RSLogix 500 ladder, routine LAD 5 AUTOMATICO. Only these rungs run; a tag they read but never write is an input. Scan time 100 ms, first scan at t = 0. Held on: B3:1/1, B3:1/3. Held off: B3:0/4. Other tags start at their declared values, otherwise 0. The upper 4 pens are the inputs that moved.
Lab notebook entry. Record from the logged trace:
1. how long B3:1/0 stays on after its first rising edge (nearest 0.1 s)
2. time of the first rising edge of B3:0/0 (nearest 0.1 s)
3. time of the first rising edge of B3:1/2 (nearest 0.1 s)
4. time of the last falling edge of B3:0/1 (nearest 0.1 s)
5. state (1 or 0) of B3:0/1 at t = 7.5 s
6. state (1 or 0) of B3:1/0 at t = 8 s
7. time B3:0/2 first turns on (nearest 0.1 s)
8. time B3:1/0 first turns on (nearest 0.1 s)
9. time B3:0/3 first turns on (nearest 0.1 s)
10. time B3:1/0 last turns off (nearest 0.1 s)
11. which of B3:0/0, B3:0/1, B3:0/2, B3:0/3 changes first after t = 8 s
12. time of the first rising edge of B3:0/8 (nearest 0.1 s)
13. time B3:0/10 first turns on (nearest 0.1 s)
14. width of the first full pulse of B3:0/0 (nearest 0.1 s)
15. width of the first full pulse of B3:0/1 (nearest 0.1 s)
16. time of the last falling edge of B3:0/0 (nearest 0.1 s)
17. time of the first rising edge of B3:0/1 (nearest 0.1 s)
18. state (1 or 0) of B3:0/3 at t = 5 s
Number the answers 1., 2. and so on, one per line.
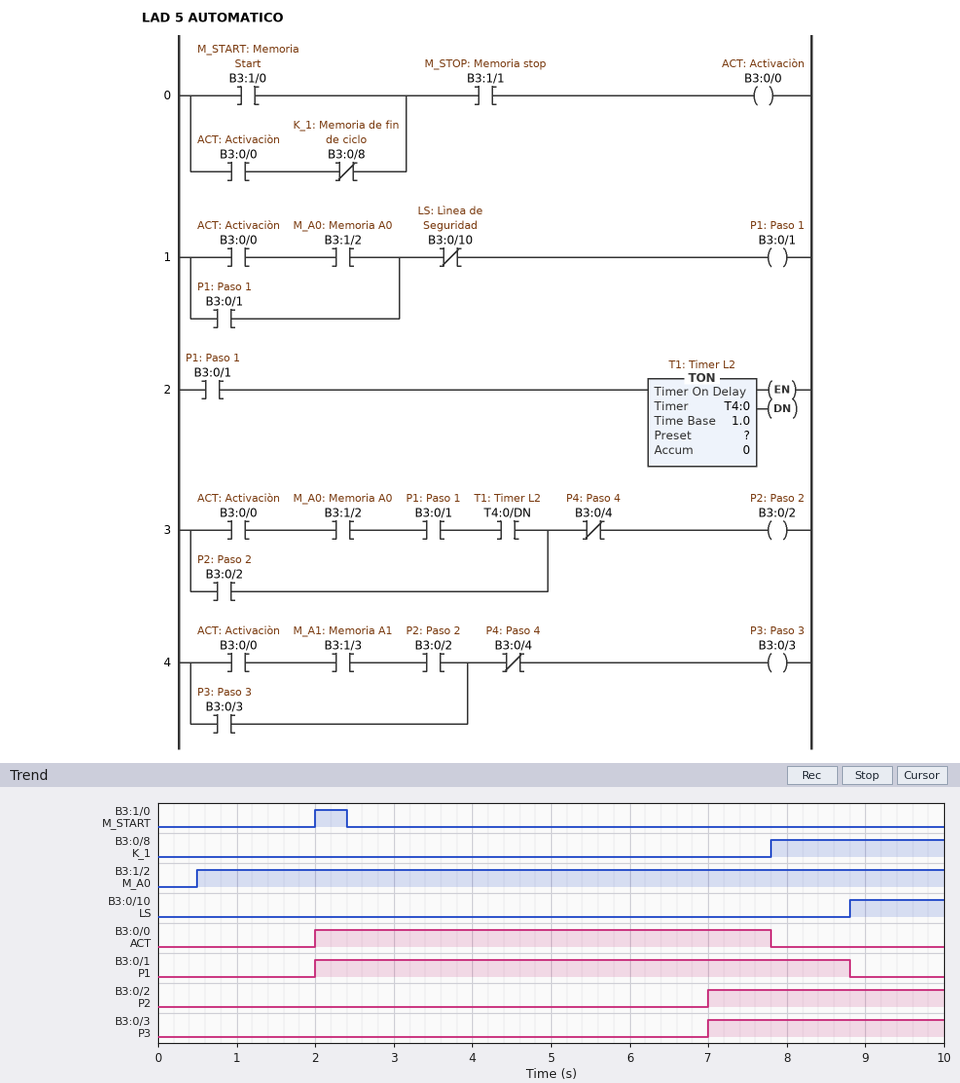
1. 0.4 s
2. 2.0 s
3. 0.5 s
4. 8.8 s
5. 1
6. 0
7. 7.0 s
8. 2.0 s
9. 7.0 s
10. 2.4 s
11. B3:0/1
12. 7.8 s
13. 8.8 s
14. 5.8 s
15. 6.8 s
16. 7.8 s
17. 2.0 s
18. 0
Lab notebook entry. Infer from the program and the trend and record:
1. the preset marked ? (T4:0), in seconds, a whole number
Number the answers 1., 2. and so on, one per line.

1. 5 s
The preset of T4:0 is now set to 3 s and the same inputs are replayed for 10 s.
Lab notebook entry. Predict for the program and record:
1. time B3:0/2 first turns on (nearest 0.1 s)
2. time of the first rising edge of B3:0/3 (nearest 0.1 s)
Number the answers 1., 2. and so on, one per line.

1. 5.0 s
2. 5.0 s
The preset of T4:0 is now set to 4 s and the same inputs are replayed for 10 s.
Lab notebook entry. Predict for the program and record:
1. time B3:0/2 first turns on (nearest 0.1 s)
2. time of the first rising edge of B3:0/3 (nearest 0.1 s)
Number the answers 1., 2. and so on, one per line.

1. 6.0 s
2. 6.0 s
